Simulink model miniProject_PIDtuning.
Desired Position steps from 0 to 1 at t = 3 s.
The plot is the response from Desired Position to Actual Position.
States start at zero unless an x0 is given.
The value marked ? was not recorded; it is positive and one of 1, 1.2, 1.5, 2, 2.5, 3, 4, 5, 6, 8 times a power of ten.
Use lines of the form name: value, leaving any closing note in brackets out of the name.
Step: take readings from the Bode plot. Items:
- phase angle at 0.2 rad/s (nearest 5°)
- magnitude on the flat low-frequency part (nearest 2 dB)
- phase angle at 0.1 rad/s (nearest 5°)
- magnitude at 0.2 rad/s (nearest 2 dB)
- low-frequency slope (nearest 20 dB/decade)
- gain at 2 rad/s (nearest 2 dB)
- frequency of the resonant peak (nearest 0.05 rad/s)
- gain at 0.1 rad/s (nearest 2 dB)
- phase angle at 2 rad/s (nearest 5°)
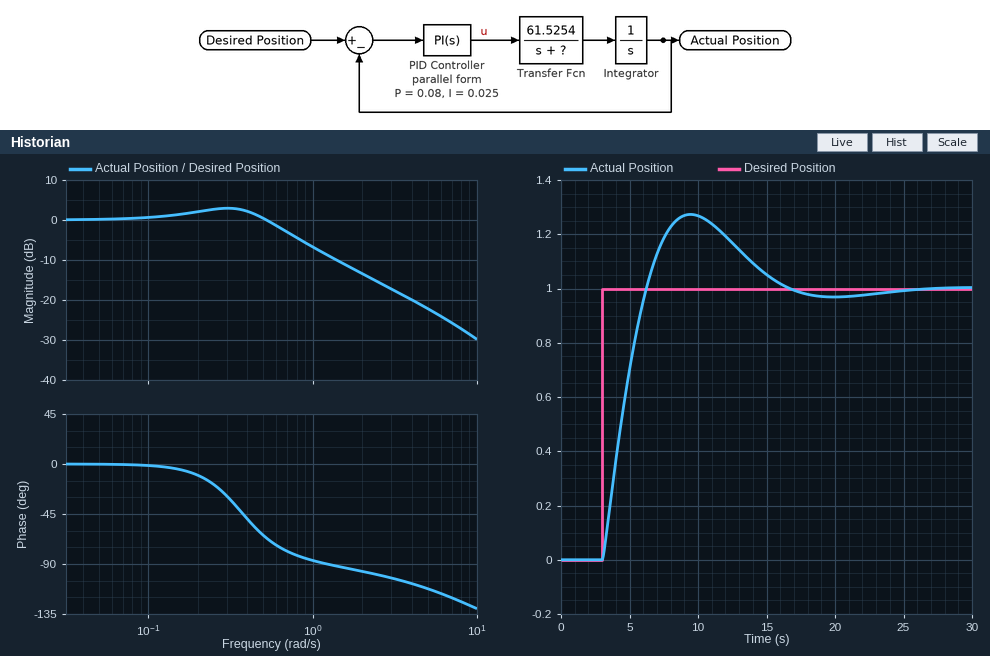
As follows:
phase angle at 0.2 rad/s: -10°
magnitude on the flat low-frequency part: 0 dB
phase angle at 0.1 rad/s: 0°
magnitude at 0.2 rad/s: 2 dB
low-frequency slope: 0 dB/decade
gain at 2 rad/s: -14 dB
frequency of the resonant peak: 0.30 rad/s
gain at 0.1 rad/s: 0 dB
phase angle at 2 rad/s: -95°
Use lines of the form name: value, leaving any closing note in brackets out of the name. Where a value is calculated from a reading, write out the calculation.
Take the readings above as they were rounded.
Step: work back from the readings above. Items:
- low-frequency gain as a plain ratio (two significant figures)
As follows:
low-frequency gain as a plain ratio: 10^(0 / 20) = 1.0
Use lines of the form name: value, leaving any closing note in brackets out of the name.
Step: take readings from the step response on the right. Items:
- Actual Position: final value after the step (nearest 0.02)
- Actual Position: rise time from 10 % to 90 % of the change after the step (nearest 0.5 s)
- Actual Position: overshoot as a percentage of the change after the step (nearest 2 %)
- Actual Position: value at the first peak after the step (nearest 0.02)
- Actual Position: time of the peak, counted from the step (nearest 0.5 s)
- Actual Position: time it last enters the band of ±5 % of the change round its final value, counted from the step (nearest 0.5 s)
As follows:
Actual Position: final value after the step: 1.00
Actual Position: rise time from 10 % to 90 % of the change after the step: 2.5 s
Actual Position: overshoot as a percentage of the change after the step: 28 %
Actual Position: value at the first peak after the step: 1.28
Actual Position: time of the peak, counted from the step: 6.5 s
Actual Position: time it last enters the band of ±5 % of the change round its final value, counted from the step: 12.0 s
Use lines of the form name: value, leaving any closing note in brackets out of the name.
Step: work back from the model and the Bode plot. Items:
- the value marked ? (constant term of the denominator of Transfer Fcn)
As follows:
the value marked ?: 12
